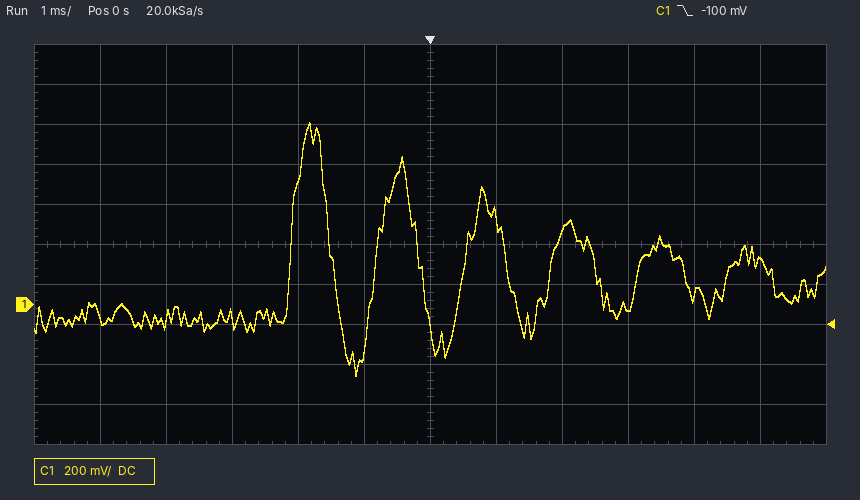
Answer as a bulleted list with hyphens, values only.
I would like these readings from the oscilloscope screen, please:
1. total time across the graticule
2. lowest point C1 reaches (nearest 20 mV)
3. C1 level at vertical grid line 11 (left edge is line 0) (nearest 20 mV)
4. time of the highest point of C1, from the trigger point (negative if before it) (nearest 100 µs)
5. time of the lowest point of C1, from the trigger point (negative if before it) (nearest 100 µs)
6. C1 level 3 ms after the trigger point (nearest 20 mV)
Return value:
- 12 ms
- -360 mV
- 220 mV
- -1.8 ms
- -1.1 ms
- -20 mV
